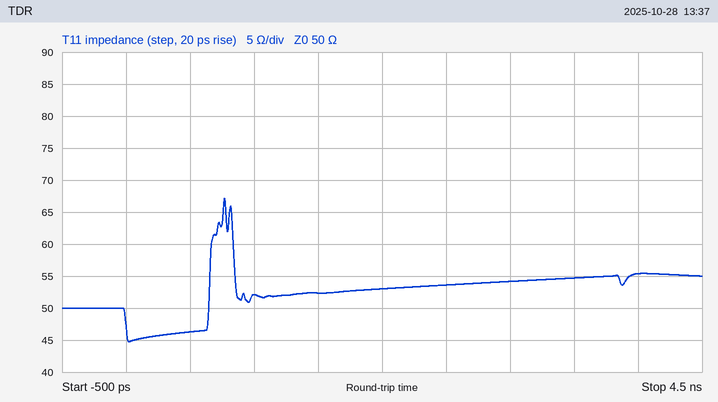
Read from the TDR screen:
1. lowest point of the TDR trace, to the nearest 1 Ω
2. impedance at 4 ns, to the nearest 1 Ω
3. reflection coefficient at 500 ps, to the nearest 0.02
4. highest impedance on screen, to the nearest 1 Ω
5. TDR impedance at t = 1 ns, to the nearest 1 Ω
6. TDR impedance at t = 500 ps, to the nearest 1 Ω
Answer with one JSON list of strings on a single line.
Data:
["45 Ω", "55 Ω", "-0.04", "67 Ω", "52 Ω", "46 Ω"]
